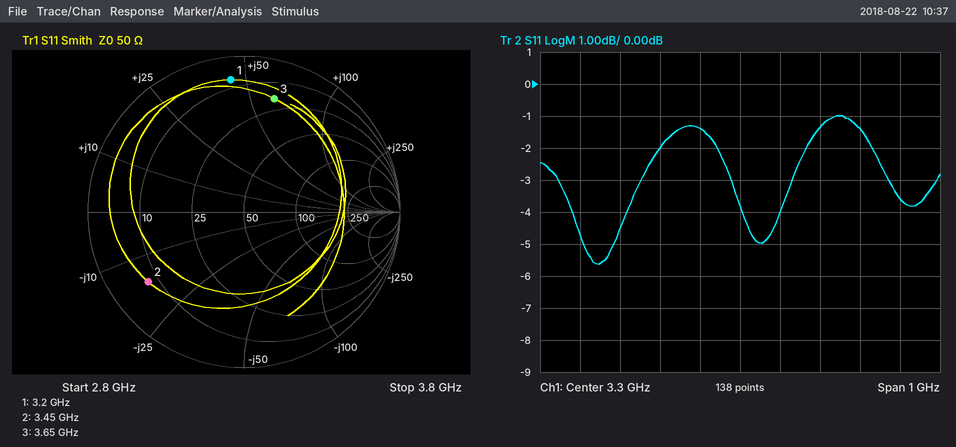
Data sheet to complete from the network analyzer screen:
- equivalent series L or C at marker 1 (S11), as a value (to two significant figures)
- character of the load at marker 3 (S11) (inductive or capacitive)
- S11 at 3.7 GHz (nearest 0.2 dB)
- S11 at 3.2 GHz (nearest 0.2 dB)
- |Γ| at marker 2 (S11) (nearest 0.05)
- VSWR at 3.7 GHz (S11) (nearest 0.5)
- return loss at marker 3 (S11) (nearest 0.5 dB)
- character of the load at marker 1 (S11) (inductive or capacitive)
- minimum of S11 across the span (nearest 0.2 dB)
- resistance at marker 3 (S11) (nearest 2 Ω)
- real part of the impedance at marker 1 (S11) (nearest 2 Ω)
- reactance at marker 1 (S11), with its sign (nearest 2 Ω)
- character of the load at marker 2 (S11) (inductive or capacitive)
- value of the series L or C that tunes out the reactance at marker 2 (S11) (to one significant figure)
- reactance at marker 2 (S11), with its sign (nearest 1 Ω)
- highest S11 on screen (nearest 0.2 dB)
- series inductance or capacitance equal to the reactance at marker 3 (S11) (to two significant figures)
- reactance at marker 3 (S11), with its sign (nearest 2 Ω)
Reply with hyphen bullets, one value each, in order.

- 2.2 nH
- inductive
- -3.6 dB
- -1.4 dB
- 0.75
- 5.0
- 2.5 dB
- inductive
- -5.6 dB
- 18 Ω
- 8 Ω
- +44 Ω
- capacitive
- 700 pH
- -16 Ω
- -1.0 dB
- 2.7 nH
- +62 Ω
